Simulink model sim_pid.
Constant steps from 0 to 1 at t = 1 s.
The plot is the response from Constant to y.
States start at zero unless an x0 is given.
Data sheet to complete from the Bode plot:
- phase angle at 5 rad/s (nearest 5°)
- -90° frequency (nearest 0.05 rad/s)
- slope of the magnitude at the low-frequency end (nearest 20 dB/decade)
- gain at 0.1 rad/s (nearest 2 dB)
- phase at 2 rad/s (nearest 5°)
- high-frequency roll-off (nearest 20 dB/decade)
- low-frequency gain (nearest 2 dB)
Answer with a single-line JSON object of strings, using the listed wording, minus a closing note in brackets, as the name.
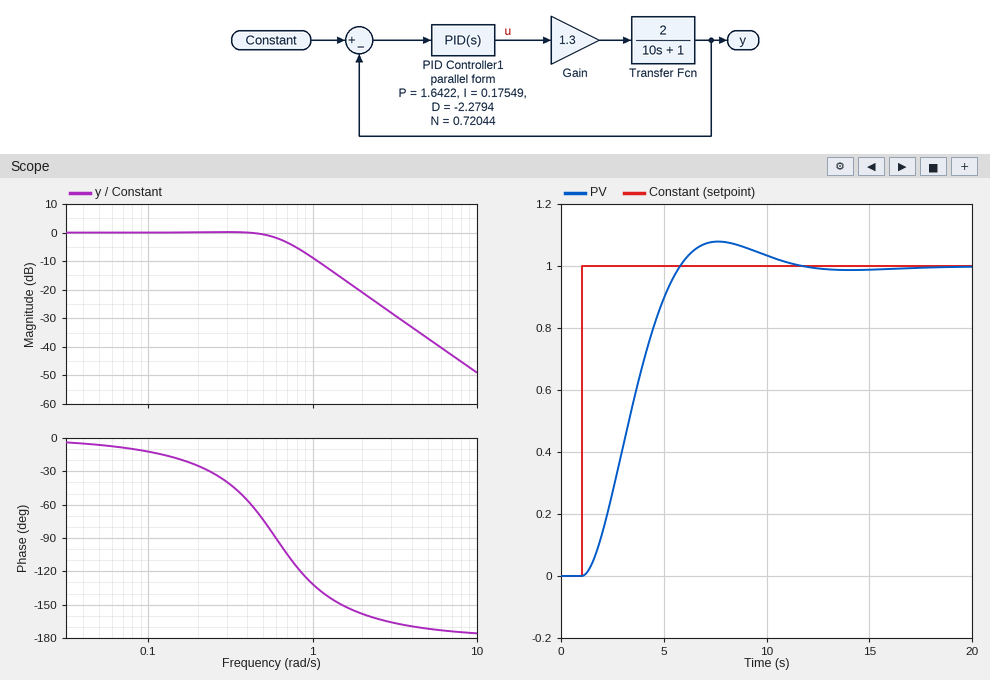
{"phase angle at 5 rad/s": "-170°", "-90° frequency": "0.60 rad/s", "slope of the magnitude at the low-frequency end": "0 dB/decade", "gain at 0.1 rad/s": "0 dB", "phase at 2 rad/s": "-160°", "high-frequency roll-off": "-40 dB/decade", "low-frequency gain": "0 dB"}
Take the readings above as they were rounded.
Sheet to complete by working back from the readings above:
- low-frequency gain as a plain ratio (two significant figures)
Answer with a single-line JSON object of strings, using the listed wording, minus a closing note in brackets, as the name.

{"low-frequency gain as a plain ratio": "1.0"}
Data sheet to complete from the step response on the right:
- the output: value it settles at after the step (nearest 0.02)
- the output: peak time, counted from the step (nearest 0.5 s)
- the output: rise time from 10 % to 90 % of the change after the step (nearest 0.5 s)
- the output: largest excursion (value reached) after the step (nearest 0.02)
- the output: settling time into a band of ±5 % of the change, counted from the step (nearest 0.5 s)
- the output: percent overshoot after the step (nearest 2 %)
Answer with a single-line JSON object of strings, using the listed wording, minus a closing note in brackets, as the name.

{"the output: value it settles at after the step": "1.00", "the output: peak time, counted from the step": "6.5 s", "the output: rise time from 10 % to 90 % of the change after the step": "3.0 s", "the output: largest excursion (value reached) after the step": "1.08", "the output: settling time into a band of ±5 % of the change, counted from the step": "8.5 s", "the output: percent overshoot after the step": "8 %"}
